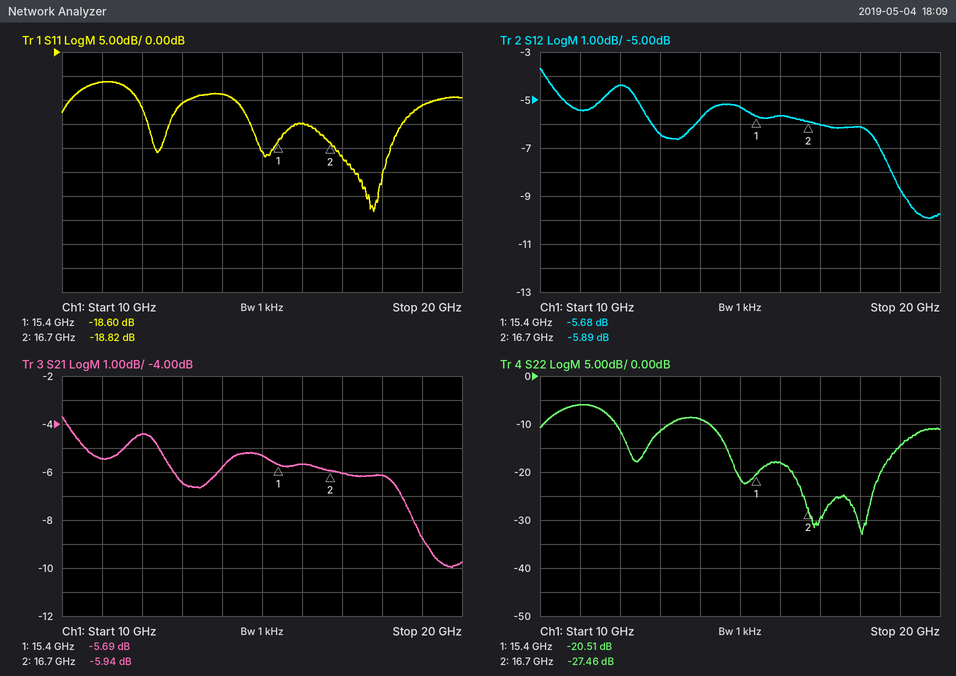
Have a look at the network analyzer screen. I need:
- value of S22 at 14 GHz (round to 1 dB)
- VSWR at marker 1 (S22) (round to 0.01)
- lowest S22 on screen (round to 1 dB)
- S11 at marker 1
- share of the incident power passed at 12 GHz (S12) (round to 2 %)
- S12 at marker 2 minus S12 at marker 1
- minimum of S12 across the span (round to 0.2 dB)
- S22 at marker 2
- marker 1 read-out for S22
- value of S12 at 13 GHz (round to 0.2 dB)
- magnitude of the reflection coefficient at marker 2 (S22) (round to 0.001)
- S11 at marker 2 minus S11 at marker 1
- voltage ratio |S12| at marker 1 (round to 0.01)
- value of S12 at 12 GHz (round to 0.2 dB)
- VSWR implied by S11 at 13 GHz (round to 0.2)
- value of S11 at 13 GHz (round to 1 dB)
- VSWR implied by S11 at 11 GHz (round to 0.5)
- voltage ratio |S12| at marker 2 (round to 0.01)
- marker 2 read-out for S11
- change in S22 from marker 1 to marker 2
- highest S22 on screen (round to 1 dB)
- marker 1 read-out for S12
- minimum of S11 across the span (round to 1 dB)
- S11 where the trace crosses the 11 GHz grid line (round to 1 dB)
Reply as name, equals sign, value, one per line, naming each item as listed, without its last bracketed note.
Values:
value of S22 at 14 GHz = -9 dB
VSWR at marker 1 (S22) = 1.21
lowest S22 on screen = -33 dB
S11 at marker 1 = -18.60 dB
share of the incident power passed at 12 GHz (S12) = 36 %
S12 at marker 2 minus S12 at marker 1 = -0.21 dB
minimum of S12 across the span = -10.0 dB
S22 at marker 2 = -27.46 dB
marker 1 read-out for S22 = -20.51 dB
value of S12 at 13 GHz = -6.4 dB
magnitude of the reflection coefficient at marker 2 (S22) = 0.042
S11 at marker 2 minus S11 at marker 1 = -0.22 dB
voltage ratio |S12| at marker 1 = 0.52
value of S12 at 12 GHz = -4.4 dB
VSWR implied by S11 at 13 GHz = 1.8
value of S11 at 13 GHz = -11 dB
VSWR implied by S11 at 11 GHz = 3.0
voltage ratio |S12| at marker 2 = 0.51
marker 2 read-out for S11 = -18.82 dB
change in S22 from marker 1 to marker 2 = -6.95 dB
highest S22 on screen = -6 dB
marker 1 read-out for S12 = -5.68 dB
minimum of S11 across the span = -33 dB
S11 where the trace crosses the 11 GHz grid line = -6 dB
